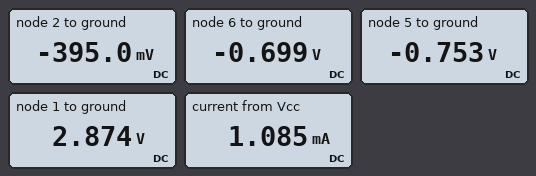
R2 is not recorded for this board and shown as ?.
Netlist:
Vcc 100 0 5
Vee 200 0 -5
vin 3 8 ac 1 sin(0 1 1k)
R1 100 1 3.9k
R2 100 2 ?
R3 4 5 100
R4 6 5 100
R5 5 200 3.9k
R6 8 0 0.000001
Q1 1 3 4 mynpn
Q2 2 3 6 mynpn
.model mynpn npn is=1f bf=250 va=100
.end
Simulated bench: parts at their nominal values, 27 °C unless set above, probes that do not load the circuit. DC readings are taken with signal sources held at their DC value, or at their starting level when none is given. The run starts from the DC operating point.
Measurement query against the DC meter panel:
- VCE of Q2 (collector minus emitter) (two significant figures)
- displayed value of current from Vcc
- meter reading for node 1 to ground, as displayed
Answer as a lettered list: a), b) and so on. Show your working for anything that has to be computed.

a) -395 mV - (-699 mV) = 300 mV
b) 1.085 mA
c) 2.874 V
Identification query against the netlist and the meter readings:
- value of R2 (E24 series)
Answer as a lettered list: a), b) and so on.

a) 10 kΩ
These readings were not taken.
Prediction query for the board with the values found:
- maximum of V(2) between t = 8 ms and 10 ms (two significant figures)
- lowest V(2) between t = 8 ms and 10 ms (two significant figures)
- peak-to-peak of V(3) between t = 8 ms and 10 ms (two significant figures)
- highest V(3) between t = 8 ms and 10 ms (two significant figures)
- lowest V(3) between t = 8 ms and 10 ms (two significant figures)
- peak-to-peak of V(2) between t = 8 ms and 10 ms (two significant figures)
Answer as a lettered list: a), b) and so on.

a) 850 mV
b) -470 mV
c) 2.0 V
d) 1.0 V
e) -1.0 V
f) 1.3 V
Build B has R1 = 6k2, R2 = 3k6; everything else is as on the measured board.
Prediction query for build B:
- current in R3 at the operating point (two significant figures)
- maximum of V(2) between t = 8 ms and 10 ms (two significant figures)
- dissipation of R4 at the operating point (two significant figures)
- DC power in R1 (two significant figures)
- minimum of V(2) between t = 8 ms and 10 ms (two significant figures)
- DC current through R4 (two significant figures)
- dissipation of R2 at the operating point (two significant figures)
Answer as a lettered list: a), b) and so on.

a) 540 µA
b) 3.5 V
c) 30 µW
d) 1.8 mW
e) 2.6 V
f) 550 µA
g) 1.1 mW
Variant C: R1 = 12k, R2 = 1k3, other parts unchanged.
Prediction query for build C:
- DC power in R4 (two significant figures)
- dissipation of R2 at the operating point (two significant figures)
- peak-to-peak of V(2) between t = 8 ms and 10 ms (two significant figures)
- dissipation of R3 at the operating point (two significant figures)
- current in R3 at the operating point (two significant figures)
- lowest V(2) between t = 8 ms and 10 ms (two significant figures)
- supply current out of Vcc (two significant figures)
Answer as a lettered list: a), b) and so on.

a) 31 µW
b) 400 µW
c) 360 mV
d) 28 µW
e) 530 µA
f) 4.1 V
g) 1.0 mA
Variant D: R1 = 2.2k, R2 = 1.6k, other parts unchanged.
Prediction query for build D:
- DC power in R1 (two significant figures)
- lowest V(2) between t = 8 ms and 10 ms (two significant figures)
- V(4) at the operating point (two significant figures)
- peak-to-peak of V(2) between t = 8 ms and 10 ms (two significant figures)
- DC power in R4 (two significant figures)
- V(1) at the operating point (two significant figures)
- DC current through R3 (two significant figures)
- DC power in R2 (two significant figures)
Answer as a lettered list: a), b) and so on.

a) 650 µW
b) 3.9 V
c) -700 mV
d) 400 mV
e) 30 µW
f) 3.8 V
g) 540 µA
h) 470 µW
